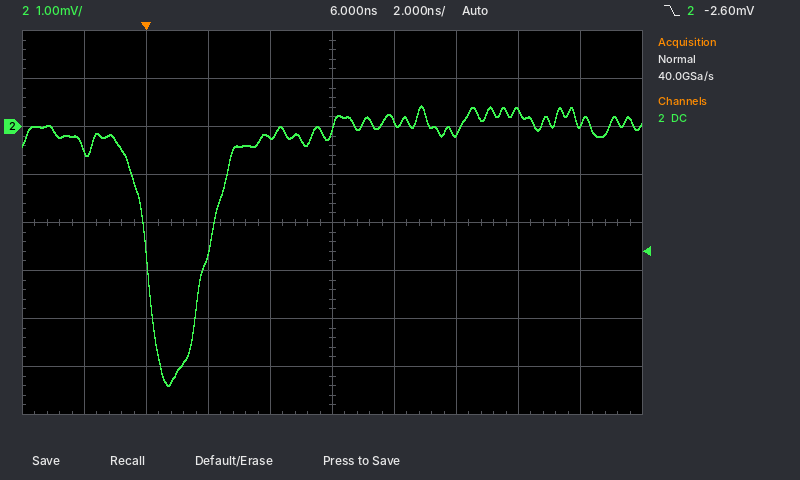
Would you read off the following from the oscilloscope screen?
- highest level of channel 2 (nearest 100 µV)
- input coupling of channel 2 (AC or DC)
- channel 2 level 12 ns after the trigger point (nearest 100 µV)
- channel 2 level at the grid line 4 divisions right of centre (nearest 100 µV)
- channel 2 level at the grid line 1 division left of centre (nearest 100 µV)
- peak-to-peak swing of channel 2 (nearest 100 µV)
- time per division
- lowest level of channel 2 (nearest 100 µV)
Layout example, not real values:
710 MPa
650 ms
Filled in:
400 µV
DC
300 µV
100 µV
-200 µV
5.8 mV
2 ns
-5.4 mV
